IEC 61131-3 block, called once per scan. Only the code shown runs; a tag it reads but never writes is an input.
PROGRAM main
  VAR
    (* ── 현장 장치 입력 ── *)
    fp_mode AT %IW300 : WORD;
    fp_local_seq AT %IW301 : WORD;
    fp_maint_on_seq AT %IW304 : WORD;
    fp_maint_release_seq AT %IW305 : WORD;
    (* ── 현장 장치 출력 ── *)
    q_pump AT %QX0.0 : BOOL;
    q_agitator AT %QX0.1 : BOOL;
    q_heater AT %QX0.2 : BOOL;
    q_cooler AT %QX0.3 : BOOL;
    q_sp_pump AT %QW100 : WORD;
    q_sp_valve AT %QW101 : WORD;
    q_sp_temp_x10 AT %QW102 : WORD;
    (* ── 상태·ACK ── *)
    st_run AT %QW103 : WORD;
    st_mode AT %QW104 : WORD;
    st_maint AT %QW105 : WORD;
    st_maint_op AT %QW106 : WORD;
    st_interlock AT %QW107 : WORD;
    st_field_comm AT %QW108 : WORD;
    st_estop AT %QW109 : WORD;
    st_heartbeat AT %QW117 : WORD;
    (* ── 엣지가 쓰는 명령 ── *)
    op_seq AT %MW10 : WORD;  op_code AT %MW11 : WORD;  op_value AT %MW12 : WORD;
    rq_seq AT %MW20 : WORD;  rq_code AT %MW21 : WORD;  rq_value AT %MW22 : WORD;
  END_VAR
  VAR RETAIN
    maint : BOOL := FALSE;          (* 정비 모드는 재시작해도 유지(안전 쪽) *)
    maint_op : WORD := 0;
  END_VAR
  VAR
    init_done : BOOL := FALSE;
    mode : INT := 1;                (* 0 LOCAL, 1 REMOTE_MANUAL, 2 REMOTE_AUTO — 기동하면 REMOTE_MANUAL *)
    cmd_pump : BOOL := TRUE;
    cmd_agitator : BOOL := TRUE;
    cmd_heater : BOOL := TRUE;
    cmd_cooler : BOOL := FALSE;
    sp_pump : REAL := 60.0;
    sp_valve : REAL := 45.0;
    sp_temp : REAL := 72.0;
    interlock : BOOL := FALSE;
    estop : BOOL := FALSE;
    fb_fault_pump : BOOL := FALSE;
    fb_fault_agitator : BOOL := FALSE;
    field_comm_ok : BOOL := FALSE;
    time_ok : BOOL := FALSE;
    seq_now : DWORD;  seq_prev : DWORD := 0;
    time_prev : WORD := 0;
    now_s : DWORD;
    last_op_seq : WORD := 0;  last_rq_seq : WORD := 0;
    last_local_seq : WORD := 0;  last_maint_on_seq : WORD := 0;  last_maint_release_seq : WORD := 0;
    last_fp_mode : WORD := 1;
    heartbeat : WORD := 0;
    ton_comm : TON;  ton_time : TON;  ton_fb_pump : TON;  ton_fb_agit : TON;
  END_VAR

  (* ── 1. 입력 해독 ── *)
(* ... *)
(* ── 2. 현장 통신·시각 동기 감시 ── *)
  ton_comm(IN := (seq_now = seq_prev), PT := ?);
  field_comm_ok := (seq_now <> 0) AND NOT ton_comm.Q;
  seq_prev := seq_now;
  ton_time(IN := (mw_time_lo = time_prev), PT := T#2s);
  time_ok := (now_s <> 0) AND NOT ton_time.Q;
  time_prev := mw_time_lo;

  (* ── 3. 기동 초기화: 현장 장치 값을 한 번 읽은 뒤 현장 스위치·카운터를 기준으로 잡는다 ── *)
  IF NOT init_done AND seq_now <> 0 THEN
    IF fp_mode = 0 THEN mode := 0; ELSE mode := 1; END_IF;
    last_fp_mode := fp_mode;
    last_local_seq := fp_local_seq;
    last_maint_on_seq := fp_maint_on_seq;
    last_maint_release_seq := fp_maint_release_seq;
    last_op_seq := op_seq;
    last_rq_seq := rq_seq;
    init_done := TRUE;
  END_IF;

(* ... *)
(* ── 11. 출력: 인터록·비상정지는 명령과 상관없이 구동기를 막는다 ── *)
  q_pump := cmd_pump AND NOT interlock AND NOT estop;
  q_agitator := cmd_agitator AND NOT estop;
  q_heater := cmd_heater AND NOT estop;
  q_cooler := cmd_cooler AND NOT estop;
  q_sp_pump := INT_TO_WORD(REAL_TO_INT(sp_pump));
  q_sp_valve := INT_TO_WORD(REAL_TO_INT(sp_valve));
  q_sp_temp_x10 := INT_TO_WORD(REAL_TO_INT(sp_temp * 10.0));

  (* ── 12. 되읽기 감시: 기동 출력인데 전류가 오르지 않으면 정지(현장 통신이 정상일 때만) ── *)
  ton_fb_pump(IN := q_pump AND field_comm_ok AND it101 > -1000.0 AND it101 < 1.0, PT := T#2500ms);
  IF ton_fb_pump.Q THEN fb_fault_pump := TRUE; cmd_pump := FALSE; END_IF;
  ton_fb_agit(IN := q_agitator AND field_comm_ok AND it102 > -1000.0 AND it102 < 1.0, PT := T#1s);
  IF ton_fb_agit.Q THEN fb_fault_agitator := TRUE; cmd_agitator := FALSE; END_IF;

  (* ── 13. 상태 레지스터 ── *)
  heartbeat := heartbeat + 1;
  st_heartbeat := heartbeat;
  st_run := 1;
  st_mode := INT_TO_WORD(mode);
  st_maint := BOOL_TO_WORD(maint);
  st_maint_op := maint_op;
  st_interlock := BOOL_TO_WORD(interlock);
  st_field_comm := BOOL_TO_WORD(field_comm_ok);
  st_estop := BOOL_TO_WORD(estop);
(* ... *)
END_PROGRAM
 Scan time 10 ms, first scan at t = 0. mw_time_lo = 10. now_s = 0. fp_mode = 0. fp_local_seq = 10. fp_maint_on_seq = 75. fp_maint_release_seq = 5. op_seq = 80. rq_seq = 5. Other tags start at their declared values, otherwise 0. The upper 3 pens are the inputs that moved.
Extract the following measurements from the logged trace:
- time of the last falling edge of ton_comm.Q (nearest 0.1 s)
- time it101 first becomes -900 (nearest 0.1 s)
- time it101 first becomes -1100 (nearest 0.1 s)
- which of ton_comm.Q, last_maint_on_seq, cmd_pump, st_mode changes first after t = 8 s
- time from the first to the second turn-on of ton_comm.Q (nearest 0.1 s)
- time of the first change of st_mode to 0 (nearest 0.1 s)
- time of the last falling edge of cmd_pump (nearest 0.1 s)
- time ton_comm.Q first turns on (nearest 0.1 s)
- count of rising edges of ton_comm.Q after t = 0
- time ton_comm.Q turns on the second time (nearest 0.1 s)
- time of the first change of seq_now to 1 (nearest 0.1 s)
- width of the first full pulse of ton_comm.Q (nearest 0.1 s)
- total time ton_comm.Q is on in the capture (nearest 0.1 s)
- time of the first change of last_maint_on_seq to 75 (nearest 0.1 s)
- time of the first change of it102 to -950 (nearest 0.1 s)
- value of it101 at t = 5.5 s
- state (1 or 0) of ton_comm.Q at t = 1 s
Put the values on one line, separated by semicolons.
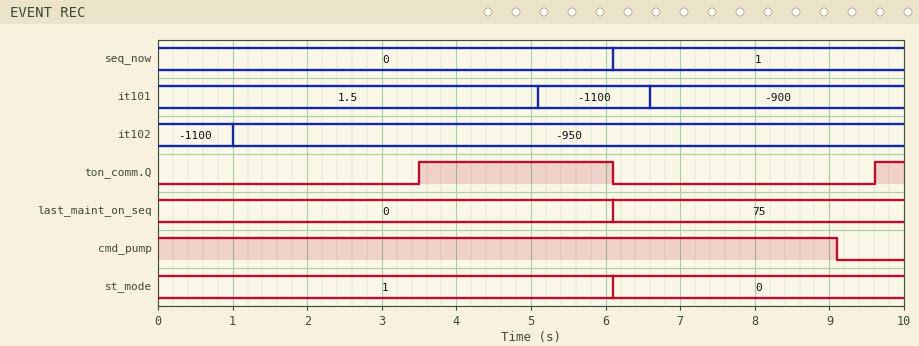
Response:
6.1 s; 6.6 s; 5.1 s; cmd_pump; 6.1 s; 6.1 s; 9.1 s; 3.5 s; 2; 9.6 s; 6.1 s; 2.6 s; 3.0 s; 6.1 s; 1.0 s; -1100; 0
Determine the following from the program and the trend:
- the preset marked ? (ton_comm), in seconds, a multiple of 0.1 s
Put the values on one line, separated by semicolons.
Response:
3.5 s
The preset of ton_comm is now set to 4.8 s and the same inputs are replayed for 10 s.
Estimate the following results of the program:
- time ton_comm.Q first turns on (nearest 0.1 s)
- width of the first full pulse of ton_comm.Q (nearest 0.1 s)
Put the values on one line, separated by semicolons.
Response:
4.8 s; 1.3 s
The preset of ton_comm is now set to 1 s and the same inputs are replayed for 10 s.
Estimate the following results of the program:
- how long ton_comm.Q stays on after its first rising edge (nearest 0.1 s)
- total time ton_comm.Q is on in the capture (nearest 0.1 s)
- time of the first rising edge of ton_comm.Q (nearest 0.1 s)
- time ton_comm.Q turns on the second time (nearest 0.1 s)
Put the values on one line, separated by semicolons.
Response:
5.1 s; 8.0 s; 1.0 s; 7.1 s
